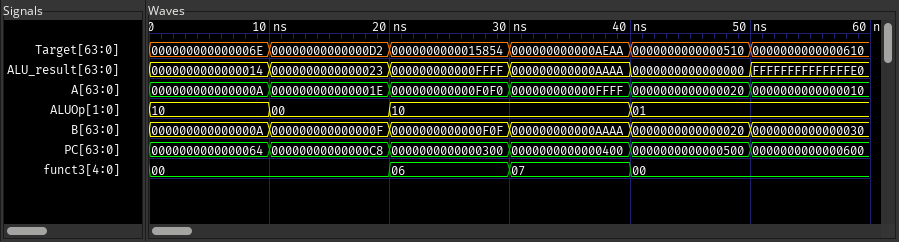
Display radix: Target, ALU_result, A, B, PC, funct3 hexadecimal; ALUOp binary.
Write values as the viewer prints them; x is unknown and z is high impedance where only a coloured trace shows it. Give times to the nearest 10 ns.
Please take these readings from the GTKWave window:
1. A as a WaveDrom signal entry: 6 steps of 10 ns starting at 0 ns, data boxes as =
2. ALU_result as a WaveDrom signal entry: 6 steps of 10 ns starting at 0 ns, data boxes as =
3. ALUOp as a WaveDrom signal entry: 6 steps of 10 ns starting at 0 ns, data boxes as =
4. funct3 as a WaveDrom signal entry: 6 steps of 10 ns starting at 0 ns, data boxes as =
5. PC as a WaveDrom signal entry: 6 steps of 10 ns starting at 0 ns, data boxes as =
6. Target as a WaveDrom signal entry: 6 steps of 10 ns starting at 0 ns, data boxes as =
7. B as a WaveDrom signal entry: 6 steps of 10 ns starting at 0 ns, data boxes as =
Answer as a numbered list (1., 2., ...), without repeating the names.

1. {name: 'A', wave: '======', data: '000000000000000A 000000000000001E 000000000000F0F0 000000000000FFFF 0000000000000020 0000000000000010'}
2. {name: 'ALU_result', wave: '======', data: '0000000000000014 0000000000000023 000000000000FFFF 000000000000AAAA 0000000000000000 FFFFFFFFFFFFFFE0'}
3. {name: 'ALUOp', wave: '===.=.', data: '10 00 10 01'}
4. {name: 'funct3', wave: '=.===.', data: '00 06 07 00'}
5. {name: 'PC', wave: '======', data: '0000000000000064 00000000000000C8 0000000000000300 0000000000000400 0000000000000500 0000000000000600'}
6. {name: 'Target', wave: '======', data: '000000000000006E 00000000000000D2 0000000000015854 000000000000AEAA 0000000000000510 0000000000000610'}
7. {name: 'B', wave: '======', data: '000000000000000A 000000000000000F 0000000000000F0F 000000000000AAAA 0000000000000020 0000000000000030'}
